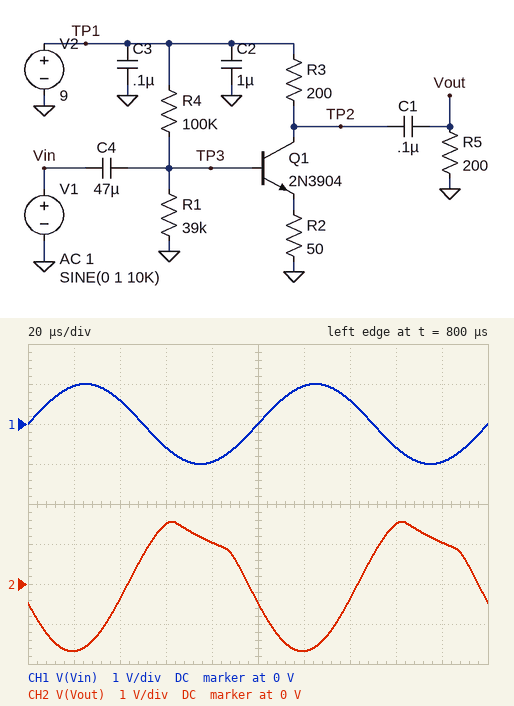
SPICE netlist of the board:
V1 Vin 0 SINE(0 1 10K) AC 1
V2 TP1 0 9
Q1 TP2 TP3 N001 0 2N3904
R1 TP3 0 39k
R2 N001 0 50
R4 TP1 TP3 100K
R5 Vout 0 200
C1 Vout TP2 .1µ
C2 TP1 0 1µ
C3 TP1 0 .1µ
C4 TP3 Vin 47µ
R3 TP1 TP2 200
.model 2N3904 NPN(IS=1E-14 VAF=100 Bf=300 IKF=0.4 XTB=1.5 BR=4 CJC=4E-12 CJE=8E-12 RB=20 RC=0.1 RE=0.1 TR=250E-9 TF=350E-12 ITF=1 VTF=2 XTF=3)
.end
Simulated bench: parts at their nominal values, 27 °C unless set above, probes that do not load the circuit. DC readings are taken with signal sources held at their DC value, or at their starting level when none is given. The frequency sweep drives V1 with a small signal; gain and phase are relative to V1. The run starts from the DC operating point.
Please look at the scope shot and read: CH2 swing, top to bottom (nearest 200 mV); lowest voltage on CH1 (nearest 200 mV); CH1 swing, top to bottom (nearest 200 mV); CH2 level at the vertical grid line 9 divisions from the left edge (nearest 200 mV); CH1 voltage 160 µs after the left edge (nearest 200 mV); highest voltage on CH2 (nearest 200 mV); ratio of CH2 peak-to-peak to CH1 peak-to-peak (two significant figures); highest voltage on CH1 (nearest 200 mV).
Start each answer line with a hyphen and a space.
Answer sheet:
- 3.2 V
- -1.0 V
- 2.0 V
- 1.0 V
- -600 mV
- 1.6 V
- 1.6
- 1.0 V
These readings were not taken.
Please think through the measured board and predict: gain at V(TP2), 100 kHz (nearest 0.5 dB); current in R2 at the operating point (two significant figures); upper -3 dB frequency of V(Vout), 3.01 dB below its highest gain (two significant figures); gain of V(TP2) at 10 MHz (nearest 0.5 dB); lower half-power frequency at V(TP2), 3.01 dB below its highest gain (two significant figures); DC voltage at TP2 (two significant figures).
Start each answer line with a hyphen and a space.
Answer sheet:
- 5.5 dB
- 13 mA
- 290 MHz
- 5.5 dB
- 340 mHz
- 6.5 V
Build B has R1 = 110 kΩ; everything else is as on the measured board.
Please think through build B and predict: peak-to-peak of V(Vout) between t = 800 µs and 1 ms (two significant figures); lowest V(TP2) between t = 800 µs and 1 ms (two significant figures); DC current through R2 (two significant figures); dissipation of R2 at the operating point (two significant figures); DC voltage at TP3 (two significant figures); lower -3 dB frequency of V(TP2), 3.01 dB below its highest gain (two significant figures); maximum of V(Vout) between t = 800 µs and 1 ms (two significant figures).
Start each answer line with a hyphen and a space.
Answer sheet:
- 3.5 V
- 3.1 V
- 18 mA
- 16 mW
- 1.6 V
- 300 mHz
- 1.7 V
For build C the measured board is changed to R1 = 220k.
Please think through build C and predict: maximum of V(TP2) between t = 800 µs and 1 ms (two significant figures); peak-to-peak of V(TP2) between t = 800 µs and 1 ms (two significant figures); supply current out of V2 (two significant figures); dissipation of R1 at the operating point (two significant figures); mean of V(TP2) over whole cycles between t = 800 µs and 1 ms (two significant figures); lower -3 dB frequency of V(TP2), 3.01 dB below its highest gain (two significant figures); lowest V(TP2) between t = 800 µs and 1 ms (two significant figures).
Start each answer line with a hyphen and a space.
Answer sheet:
- 7.3 V
- 4.5 V
- 19 mA
- 13 µW
- 5.1 V
- 290 mHz
- 2.8 V
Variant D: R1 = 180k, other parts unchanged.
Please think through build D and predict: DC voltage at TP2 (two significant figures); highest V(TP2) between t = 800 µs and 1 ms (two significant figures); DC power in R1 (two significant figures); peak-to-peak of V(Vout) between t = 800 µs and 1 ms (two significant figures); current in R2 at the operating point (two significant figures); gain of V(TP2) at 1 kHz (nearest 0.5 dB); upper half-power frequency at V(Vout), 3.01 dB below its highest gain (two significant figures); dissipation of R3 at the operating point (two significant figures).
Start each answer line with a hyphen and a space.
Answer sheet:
- 5.2 V
- 7.4 V
- 16 µW
- 3.5 V
- 19 mA
- 11.5 dB
- 280 MHz
- 72 mW
